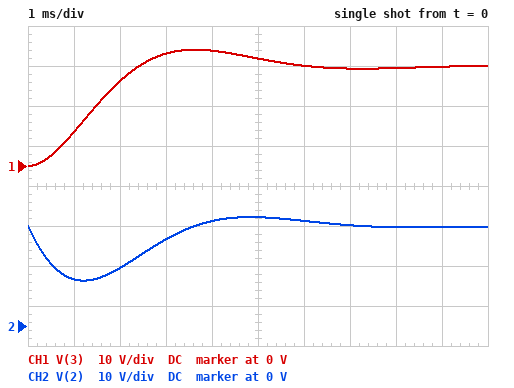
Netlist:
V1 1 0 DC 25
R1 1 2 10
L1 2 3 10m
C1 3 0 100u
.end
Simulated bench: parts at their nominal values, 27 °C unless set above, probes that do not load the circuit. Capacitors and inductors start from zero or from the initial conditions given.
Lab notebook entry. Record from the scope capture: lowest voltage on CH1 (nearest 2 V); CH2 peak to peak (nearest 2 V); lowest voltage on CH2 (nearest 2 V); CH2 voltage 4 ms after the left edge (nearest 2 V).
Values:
0 V
16 V
12 V
26 V
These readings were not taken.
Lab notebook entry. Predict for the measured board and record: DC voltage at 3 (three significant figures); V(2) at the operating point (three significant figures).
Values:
25.0 V
25.0 V
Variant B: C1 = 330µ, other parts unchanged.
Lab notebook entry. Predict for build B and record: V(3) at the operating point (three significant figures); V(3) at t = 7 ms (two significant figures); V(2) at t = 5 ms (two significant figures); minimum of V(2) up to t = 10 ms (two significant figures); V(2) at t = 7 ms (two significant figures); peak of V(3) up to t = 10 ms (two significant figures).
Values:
25.0 V
23 V
17 V
7.2 V
22 V
25 V
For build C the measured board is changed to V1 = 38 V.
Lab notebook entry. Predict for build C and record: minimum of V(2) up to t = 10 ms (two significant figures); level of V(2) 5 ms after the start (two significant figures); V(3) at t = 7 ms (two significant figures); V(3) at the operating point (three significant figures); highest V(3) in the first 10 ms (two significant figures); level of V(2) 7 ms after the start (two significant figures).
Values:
17 V
41 V
37 V
38.0 V
44 V
38 V
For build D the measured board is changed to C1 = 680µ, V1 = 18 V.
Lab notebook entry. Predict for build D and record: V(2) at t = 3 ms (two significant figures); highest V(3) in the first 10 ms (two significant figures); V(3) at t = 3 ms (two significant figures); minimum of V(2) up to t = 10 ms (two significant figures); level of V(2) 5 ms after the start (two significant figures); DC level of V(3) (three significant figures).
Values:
4.0 V
14 V
5.0 V
3.7 V
7.0 V
18.0 V
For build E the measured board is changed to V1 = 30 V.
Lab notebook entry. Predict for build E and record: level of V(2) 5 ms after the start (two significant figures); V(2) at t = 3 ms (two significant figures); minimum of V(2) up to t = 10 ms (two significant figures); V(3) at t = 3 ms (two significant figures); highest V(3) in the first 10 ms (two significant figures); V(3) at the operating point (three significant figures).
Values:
33 V
26 V
14 V
34 V
35 V
30.0 V
